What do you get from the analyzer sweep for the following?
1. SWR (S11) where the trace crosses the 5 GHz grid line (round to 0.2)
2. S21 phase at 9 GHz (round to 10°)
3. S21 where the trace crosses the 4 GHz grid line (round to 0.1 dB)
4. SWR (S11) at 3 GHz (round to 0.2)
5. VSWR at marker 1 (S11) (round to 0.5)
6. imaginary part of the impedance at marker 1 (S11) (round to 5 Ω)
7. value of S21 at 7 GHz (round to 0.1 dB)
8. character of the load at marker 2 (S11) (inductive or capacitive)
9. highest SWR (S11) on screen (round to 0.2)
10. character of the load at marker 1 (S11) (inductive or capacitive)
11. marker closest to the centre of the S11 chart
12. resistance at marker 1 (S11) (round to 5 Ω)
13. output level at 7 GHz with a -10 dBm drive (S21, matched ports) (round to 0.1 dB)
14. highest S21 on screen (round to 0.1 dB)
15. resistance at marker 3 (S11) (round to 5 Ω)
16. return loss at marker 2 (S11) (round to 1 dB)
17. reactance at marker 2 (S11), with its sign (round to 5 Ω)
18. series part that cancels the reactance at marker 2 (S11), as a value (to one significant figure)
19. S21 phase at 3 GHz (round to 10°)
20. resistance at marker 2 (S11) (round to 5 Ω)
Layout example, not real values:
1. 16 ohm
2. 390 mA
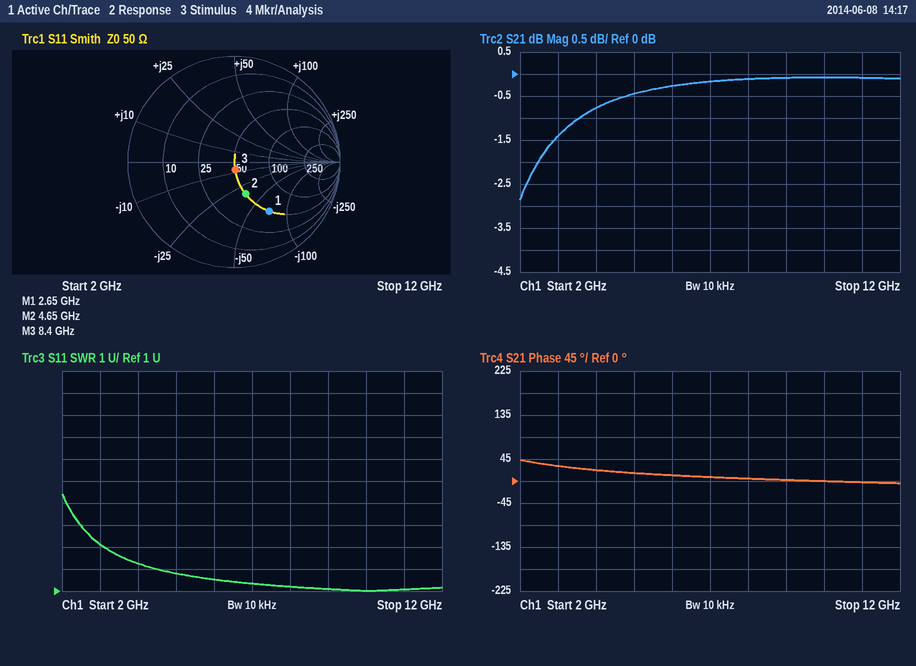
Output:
1. 1.8
2. 0°
3. -0.8 dB
4. 3.2
5. 3.5
6. -70 Ω
7. -0.2 dB
8. capacitive
9. 5.4
10. capacitive
11. marker 3
12. 50 Ω
13. -10.2 dBm
14. -0.1 dB
15. 50 Ω
16. 10 dB
17. -35 Ω
18. 1 nH
19. 30°
20. 50 Ω
